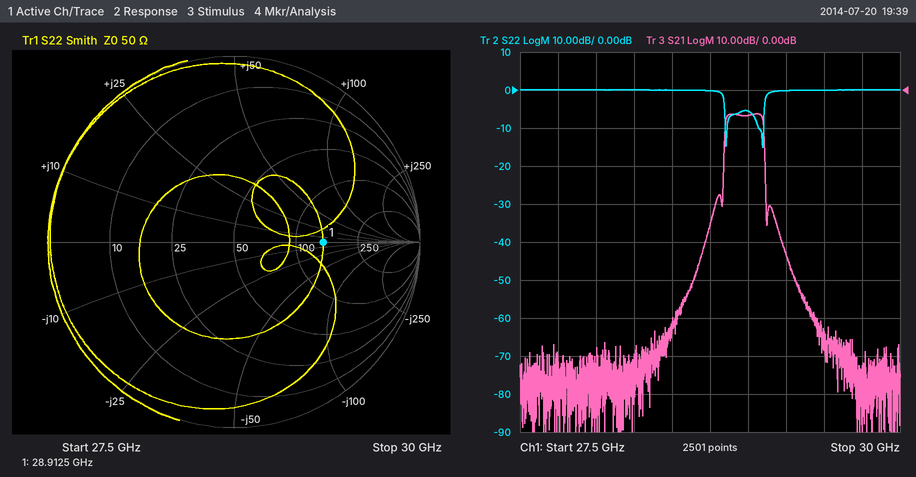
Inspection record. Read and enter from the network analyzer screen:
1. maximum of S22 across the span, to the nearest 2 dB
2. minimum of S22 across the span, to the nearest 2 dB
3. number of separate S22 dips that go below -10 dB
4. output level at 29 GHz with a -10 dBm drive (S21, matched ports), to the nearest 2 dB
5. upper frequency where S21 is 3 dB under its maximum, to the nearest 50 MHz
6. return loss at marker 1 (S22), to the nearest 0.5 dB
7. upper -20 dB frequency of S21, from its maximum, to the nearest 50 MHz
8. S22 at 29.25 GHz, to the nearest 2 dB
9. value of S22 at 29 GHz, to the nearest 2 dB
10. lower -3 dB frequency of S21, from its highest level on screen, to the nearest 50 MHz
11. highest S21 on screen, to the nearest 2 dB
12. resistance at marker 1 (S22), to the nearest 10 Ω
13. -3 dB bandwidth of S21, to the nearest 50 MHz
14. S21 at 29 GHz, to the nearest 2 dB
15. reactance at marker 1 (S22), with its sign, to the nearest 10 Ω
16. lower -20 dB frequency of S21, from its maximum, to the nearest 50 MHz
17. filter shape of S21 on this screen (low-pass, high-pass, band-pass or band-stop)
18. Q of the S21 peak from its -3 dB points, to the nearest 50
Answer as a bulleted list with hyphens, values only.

- 0 dB
- -16 dB
- 2
- -16 dBm
- 29.10 GHz
- 6.5 dB
- 29.10 GHz
- 0 dB
- -6 dB
- 28.85 GHz
- -6 dB
- 140 Ω
- 250 MHz
- -6 dB
- 0 Ω
- 28.85 GHz
- band-pass
- 100
